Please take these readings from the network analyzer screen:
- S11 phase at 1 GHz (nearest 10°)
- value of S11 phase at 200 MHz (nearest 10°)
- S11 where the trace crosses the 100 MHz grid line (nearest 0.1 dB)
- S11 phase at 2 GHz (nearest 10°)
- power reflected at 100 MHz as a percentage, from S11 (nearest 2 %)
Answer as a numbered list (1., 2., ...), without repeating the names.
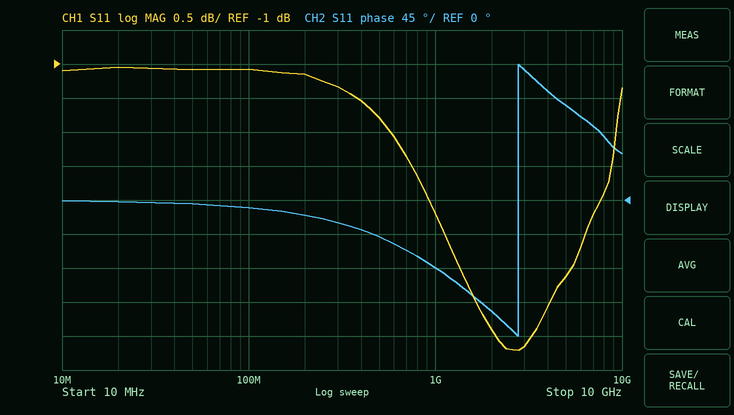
1. -90°
2. -20°
3. -1.1 dB
4. -150°
5. 78 %
